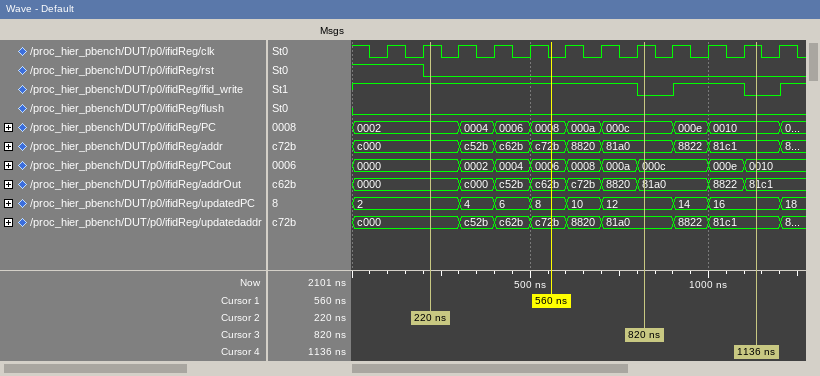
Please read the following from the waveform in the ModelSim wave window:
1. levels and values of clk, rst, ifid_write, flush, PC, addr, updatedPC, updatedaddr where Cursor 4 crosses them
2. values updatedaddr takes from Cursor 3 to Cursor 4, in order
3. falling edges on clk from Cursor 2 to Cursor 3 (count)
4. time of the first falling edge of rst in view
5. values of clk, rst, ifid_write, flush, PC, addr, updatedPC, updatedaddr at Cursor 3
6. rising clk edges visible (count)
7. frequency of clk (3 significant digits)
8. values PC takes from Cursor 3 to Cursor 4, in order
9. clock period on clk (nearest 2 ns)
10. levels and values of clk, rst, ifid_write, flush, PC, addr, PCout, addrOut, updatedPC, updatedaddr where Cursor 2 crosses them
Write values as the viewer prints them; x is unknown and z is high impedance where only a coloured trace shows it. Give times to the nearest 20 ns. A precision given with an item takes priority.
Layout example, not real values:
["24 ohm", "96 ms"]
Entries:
["clk=1, rst=0, ifid_write=0, flush=0, PC=0010, addr=81c1, updatedPC=16, updatedaddr=81c1", "81a0, 8822, 81c1", "6", "200 ns", "clk=1, rst=0, ifid_write=0, flush=0, PC=000c, addr=81a0, updatedPC=12, updatedaddr=81a0", "12", "10.0 MHz", "000c, 000e, 0010", "100 ns", "clk=1, rst=0, ifid_write=1, flush=0, PC=0002, addr=c000, PCout=0000, addrOut=0000, updatedPC=2, updatedaddr=c000"]
